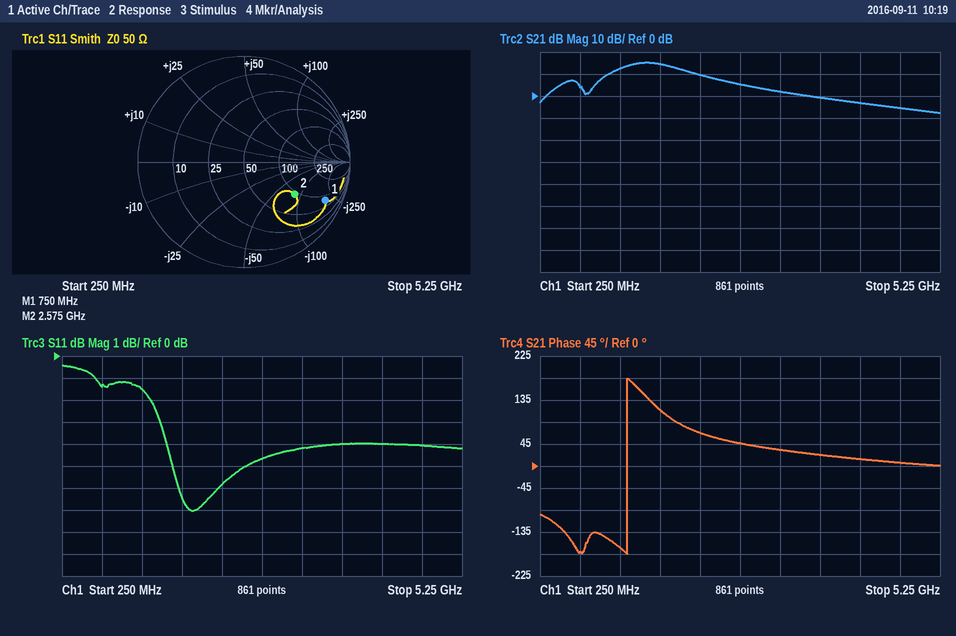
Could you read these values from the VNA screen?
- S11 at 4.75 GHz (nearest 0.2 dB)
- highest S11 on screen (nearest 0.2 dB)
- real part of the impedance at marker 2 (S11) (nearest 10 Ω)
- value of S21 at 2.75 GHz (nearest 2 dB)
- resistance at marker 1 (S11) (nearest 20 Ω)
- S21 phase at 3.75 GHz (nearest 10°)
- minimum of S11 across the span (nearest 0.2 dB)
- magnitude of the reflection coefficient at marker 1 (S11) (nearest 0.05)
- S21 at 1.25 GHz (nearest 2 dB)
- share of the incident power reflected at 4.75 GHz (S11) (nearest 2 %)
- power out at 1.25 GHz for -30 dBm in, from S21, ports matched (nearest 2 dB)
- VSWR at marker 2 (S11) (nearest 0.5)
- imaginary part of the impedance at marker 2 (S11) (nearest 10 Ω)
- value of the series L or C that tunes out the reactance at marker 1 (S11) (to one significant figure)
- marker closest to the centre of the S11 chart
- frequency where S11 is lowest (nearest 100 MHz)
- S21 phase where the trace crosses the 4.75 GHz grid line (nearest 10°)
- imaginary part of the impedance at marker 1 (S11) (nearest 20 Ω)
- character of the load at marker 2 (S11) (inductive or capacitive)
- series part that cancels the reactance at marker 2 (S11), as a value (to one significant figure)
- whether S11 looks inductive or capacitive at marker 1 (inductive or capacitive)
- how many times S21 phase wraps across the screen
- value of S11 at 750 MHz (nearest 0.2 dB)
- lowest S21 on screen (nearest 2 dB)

-4.0 dB
-0.4 dB
90 Ω
6 dB
80 Ω
20°
-7.0 dB
0.85
12 dB
40 %
-18 dBm
3.5
-80 Ω
40 nH
marker 2
1.9 GHz
10°
-200 Ω
capacitive
5 nH
capacitive
1
-1.4 dB
-8 dB
